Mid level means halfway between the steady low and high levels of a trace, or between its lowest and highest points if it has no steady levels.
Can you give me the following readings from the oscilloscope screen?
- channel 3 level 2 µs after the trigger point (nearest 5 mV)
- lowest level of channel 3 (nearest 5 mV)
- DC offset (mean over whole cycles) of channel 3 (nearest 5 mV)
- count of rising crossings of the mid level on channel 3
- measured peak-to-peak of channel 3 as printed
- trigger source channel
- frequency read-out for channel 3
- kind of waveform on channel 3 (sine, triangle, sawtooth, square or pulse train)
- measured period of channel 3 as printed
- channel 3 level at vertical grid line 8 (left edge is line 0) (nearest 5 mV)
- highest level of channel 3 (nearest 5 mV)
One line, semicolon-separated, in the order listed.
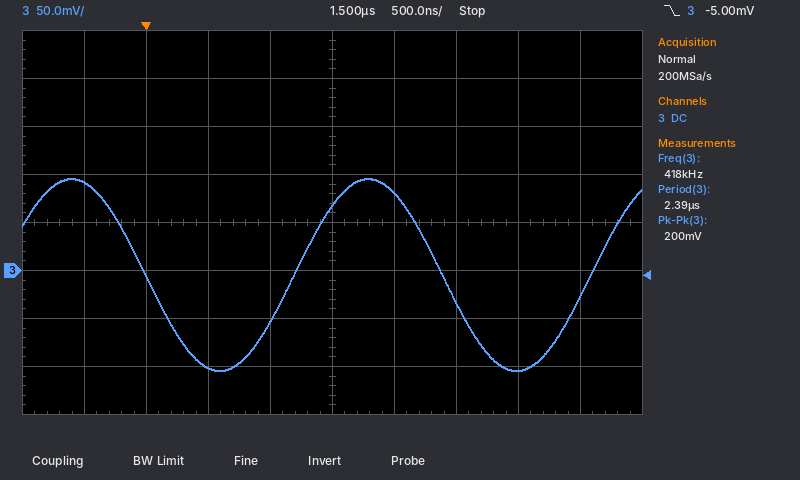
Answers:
80 mV; -105 mV; -5 mV; 2; 200 mV; channel 3; 418 kHz; sine; 2.39 µs; -105 mV; 95 mV
